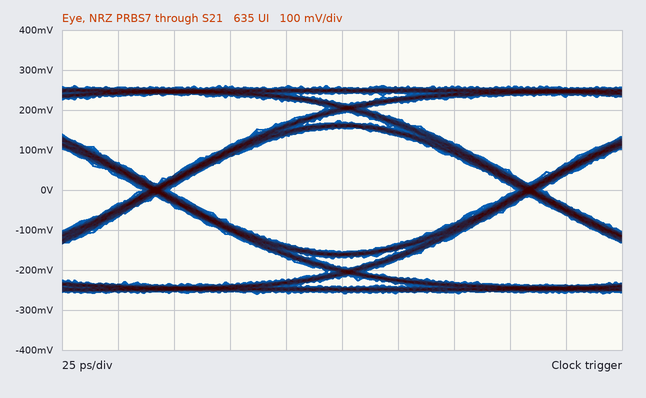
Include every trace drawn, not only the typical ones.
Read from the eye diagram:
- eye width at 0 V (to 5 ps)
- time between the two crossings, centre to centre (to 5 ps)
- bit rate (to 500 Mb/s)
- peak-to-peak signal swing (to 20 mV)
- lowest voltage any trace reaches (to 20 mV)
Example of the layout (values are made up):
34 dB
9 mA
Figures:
155 ps
165 ps
6.0 Gb/s
520 mV
-260 mV
